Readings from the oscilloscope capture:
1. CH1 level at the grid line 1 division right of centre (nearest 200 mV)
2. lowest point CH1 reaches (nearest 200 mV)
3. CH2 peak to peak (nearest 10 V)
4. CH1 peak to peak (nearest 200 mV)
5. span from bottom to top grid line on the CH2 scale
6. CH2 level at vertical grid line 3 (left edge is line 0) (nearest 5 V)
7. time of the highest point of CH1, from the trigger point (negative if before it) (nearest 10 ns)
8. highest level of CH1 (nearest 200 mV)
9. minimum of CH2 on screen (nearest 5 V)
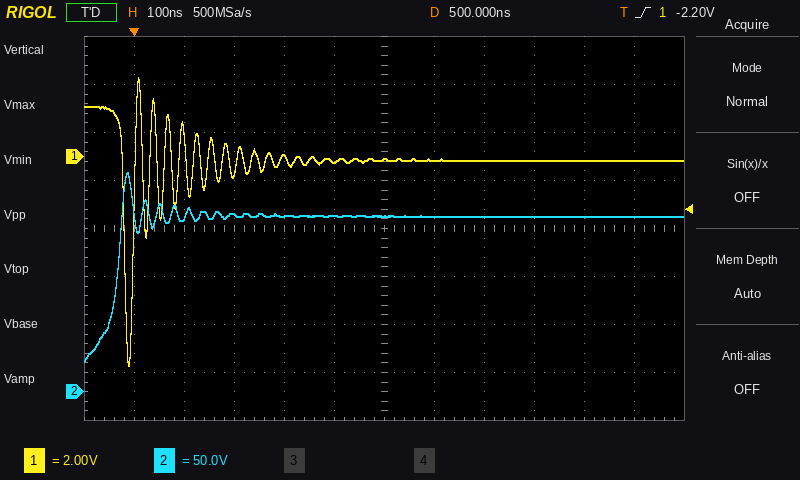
-200 mV
-8.8 V
200 V
12.0 V
400 V
185 V
+10 ns
3.2 V
30 V
